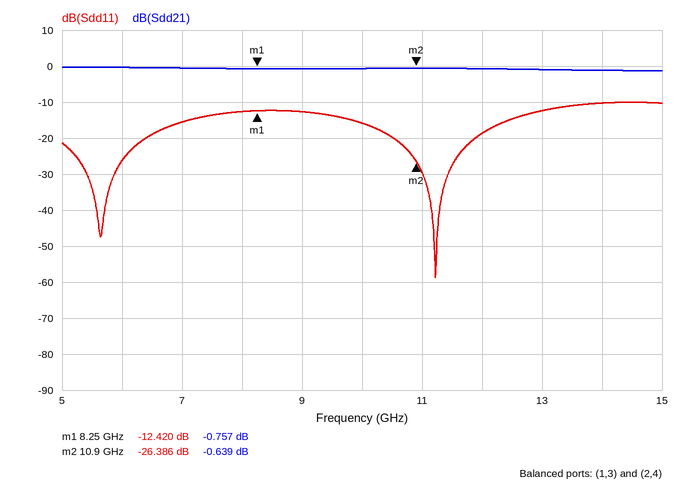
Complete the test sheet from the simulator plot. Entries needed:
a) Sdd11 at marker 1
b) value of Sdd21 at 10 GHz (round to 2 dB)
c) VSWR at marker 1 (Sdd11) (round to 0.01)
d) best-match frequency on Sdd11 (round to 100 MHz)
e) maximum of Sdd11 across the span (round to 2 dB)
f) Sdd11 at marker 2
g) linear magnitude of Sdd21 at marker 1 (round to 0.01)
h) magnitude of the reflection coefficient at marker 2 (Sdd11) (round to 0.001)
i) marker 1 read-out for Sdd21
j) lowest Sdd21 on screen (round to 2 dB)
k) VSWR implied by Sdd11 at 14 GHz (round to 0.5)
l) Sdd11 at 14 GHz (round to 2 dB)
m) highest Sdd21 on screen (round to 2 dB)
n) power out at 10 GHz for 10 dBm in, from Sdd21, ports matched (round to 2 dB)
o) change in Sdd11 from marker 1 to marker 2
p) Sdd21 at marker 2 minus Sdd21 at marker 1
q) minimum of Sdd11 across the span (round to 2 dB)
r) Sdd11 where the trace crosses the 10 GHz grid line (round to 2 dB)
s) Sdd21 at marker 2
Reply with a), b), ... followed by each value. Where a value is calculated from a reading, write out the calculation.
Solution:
a) -12.420 dB
b) 0 dB
c) (1 + 0.2393)/(1 − 0.2393) ≈ 1.63
d) 11.2 GHz
e) -10 dB
f) -26.386 dB
g) 10^(-0.757/20) ≈ 0.92
h) 10^(-26.386/20) ≈ 0.048
i) -0.757 dB
j) -2 dB
k) |Γ| = 10^(-10/20) = 0.3162; VSWR = (1 + 0.3162)/(1 − 0.3162) ≈ 1.92, so 2.0 to the nearest 0.5
l) -10 dB
m) 0 dB
n) 10 dBm + (0 dB) = 10 dBm
o) -26.386 − (-12.42) = -13.966 dB
p) -0.639 − (-0.757) = 0.118 dB
q) -58 dB
r) -16 dB
s) -0.639 dB
